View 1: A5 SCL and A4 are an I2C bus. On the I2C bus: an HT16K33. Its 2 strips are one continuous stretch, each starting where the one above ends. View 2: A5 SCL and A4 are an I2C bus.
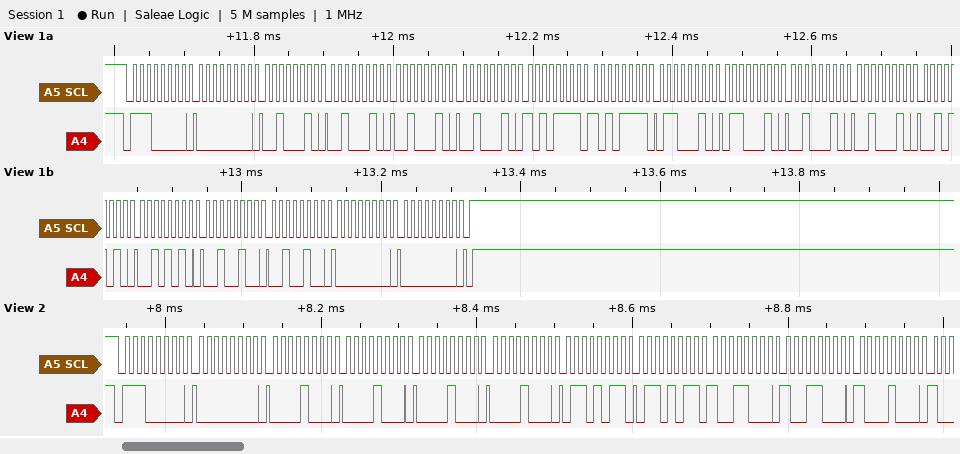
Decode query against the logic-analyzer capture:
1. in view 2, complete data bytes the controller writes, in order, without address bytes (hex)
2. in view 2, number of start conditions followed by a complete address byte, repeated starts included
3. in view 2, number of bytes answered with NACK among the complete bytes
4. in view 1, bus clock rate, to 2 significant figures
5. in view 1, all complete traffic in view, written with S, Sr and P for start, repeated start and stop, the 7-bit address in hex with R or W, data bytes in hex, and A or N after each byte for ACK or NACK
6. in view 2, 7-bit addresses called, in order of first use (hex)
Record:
00 08 08 08 08 6B 6B 98 98 88
1
0
100 kHz
S 70W A 00 A 22 A 22 A 22 A 22 A AF A AF A 62 A 62 A 22 A 22 A 2A A 2A A 24 A 24 A 00 A 00 A P
0x70
